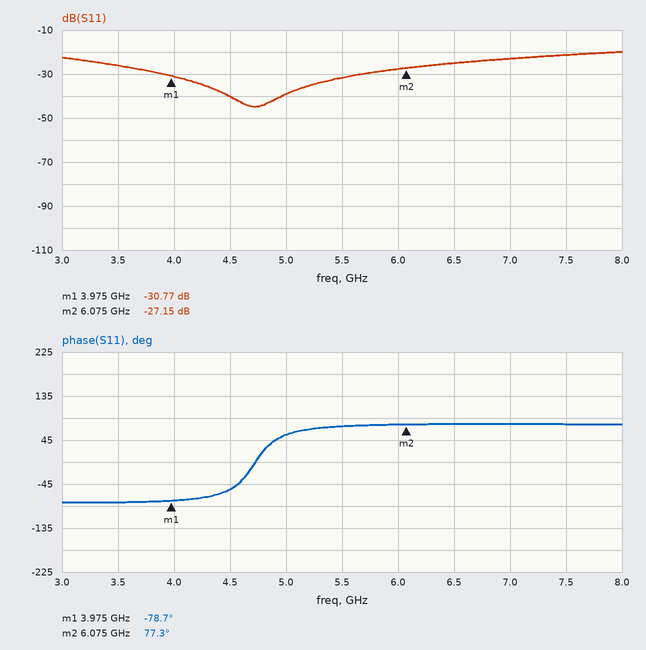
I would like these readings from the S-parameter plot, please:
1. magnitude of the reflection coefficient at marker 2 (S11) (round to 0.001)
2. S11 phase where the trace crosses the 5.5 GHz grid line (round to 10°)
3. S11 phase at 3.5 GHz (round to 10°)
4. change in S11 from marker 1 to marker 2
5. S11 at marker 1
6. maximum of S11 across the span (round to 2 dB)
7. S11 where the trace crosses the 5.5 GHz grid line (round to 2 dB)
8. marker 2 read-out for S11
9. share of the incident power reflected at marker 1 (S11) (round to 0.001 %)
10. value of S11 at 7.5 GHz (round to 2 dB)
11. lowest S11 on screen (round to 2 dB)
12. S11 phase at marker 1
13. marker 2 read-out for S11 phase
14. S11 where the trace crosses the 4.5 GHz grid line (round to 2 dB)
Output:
0.044
70°
-80°
3.62 dB
-30.77 dB
-20 dB
-32 dB
-27.15 dB
0.084 %
-22 dB
-44 dB
-78.7°
77.3°
-40 dB
